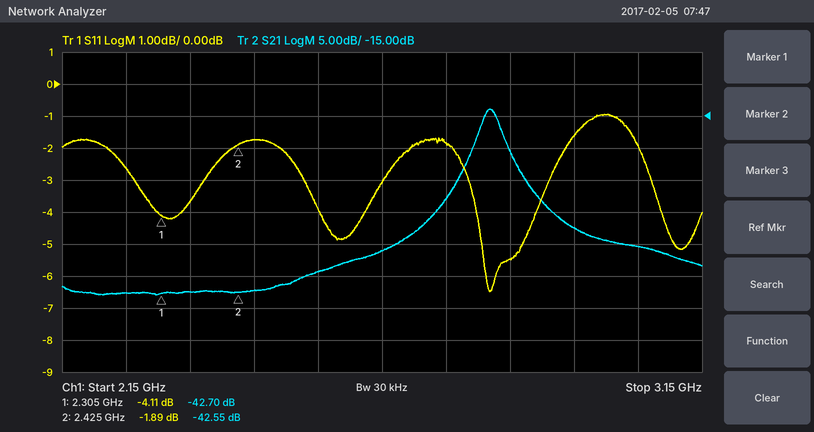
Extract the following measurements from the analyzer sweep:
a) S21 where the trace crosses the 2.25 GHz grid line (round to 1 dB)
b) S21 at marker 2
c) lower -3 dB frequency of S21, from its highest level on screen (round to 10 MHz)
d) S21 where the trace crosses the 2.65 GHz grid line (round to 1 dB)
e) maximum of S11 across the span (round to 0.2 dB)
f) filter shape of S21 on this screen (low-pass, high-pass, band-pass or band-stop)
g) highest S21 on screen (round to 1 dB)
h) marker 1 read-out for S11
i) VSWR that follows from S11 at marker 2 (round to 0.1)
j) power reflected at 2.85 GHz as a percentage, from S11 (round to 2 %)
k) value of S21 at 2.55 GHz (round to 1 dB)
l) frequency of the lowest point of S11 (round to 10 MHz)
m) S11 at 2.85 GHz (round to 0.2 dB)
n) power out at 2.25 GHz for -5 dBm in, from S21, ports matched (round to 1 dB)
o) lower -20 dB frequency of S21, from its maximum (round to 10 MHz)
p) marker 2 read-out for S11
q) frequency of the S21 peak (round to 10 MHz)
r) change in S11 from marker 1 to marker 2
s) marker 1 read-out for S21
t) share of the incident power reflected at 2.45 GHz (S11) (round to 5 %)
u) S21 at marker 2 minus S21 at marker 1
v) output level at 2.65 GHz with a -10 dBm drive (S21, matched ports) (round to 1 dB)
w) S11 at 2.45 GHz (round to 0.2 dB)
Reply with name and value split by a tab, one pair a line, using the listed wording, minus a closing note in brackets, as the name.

S21 where the trace crosses the 2.25 GHz grid line	-43 dB
S21 at marker 2	-42.55 dB
lower -3 dB frequency of S21, from its highest level on screen	2.80 GHz
S21 where the trace crosses the 2.65 GHz grid line	-36 dB
maximum of S11 across the span	-1.0 dB
filter shape of S21 on this screen	band-pass
highest S21 on screen	-14 dB
marker 1 read-out for S11	-4.11 dB
VSWR that follows from S11 at marker 2	9.2
power reflected at 2.85 GHz as a percentage, from S11	28 %
value of S21 at 2.55 GHz	-39 dB
frequency of the lowest point of S11	2.82 GHz
S11 at 2.85 GHz	-5.4 dB
power out at 2.25 GHz for -5 dBm in, from S21, ports matched	-48 dBm
lower -20 dB frequency of S21, from its maximum	2.69 GHz
marker 2 read-out for S11	-1.89 dB
frequency of the S21 peak	2.82 GHz
change in S11 from marker 1 to marker 2	2.22 dB
marker 1 read-out for S21	-42.70 dB
share of the incident power reflected at 2.45 GHz (S11)	65 %
S21 at marker 2 minus S21 at marker 1	0.15 dB
output level at 2.65 GHz with a -10 dBm drive (S21, matched ports)	-46 dBm
S11 at 2.45 GHz	-1.8 dB
